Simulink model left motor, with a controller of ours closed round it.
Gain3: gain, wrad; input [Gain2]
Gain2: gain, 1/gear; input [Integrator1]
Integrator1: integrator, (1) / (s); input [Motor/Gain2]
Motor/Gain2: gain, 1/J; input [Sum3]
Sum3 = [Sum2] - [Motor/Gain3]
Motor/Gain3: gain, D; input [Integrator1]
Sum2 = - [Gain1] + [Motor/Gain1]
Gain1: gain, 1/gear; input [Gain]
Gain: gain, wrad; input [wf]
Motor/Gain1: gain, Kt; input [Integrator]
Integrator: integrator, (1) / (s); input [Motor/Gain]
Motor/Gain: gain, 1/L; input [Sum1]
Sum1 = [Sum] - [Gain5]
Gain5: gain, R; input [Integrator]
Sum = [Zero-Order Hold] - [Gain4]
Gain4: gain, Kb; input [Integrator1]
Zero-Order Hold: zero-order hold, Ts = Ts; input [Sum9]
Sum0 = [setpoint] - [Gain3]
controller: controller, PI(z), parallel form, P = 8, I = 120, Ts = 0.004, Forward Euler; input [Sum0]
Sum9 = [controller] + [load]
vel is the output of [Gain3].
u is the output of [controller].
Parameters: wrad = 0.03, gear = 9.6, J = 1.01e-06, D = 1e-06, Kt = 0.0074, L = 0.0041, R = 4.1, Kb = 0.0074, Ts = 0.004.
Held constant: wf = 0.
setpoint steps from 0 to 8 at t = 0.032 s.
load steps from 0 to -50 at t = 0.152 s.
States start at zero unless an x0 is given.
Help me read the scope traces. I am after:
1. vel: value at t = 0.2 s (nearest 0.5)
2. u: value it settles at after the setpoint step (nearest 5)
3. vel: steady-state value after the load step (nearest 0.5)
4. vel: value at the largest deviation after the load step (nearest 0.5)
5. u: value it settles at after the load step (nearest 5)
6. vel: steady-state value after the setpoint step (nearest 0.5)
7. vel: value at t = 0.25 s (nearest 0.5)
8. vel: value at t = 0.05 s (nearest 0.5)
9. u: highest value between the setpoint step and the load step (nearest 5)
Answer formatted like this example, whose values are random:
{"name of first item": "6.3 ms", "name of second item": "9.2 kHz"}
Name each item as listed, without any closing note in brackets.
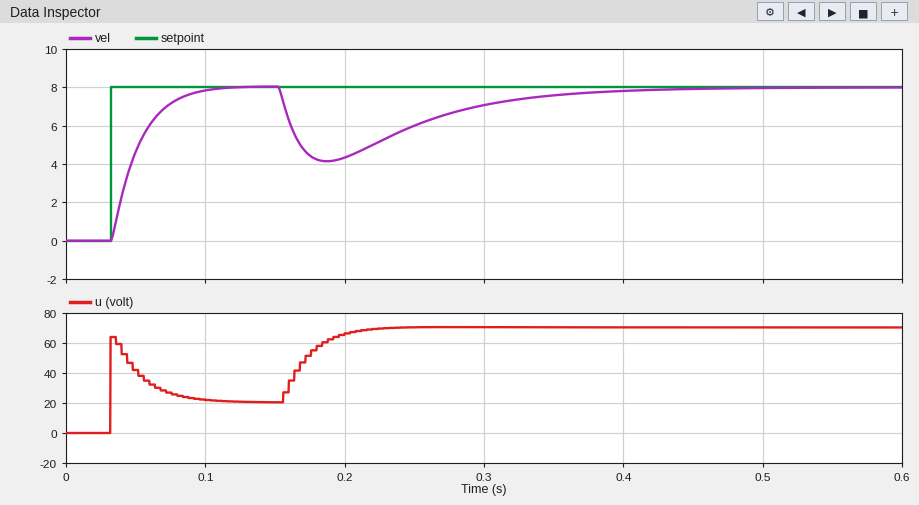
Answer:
{"vel: value at t = 0.2 s": "4.5", "u: value it settles at after the setpoint step": "20", "vel: steady-state value after the load step": "8.0", "vel: value at the largest deviation after the load step": "4.0", "u: value it settles at after the load step": "70", "vel: steady-state value after the setpoint step": "8.0", "vel: value at t = 0.25 s": "6.0", "vel: value at t = 0.05 s": "4.5", "u: highest value between the setpoint step and the load step": "65"}
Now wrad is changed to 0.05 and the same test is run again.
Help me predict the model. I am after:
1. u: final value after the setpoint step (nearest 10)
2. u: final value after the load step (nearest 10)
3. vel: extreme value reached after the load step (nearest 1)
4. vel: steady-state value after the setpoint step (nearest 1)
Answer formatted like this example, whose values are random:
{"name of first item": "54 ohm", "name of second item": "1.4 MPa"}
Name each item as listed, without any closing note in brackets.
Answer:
{"u: final value after the setpoint step": "10", "u: final value after the load step": "60", "vel: extreme value reached after the load step": "3", "vel: steady-state value after the setpoint step": "8"}
